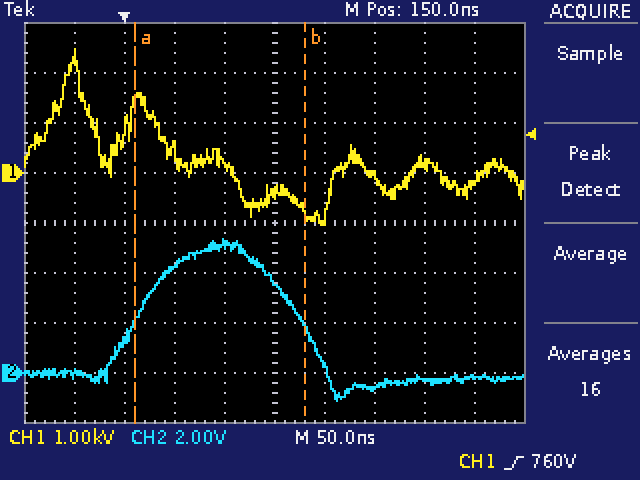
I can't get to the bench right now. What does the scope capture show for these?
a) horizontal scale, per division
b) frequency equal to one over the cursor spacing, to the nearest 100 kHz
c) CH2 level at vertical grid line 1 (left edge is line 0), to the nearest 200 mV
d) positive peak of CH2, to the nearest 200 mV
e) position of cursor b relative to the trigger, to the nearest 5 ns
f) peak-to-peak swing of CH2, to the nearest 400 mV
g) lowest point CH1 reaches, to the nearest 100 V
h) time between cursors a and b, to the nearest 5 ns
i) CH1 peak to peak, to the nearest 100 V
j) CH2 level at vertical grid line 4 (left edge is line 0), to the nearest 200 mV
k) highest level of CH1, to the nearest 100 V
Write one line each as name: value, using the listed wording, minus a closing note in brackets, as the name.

horizontal scale, per division: 50 ns
frequency equal to one over the cursor spacing, to the nearest 100 kHz: 5.9 MHz
CH2 level at vertical grid line 1 (left edge is line 0), to the nearest 200 mV: 0.0 V
positive peak of CH2, to the nearest 200 mV: 5.4 V
position of cursor b relative to the trigger, to the nearest 5 ns: +180 ns
peak-to-peak swing of CH2, to the nearest 400 mV: 6.4 V
lowest point CH1 reaches, to the nearest 100 V: -1.0 kV
time between cursors a and b, to the nearest 5 ns: 170 ns
CH1 peak to peak, to the nearest 100 V: 3.5 kV
CH2 level at vertical grid line 4 (left edge is line 0), to the nearest 200 mV: 5.2 V
highest level of CH1, to the nearest 100 V: 2.5 kV
